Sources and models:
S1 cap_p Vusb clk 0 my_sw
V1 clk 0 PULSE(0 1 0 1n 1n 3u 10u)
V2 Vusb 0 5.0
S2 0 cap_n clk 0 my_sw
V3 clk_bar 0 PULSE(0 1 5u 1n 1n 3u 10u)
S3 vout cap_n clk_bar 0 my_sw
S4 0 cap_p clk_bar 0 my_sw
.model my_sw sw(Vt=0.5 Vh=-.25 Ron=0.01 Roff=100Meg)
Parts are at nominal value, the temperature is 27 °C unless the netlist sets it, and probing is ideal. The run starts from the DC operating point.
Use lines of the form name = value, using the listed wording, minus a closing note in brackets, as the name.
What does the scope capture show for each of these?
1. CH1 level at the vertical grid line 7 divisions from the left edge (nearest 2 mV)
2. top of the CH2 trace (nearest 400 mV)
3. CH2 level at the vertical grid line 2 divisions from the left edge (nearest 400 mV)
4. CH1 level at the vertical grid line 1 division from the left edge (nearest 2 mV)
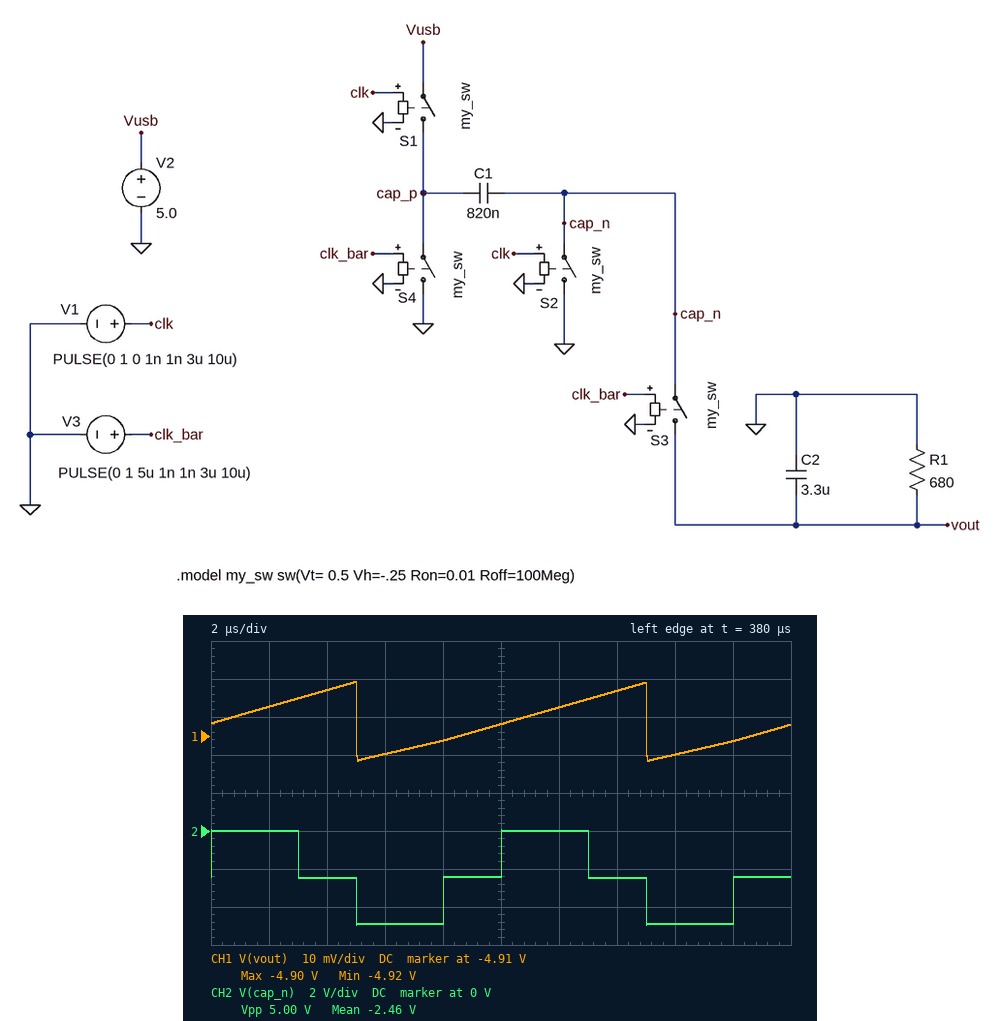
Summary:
CH1 level at the vertical grid line 7 divisions from the left edge = -4.898 V
top of the CH2 trace = 0 V
CH2 level at the vertical grid line 2 divisions from the left edge = -2.4 V
CH1 level at the vertical grid line 1 division from the left edge = -4.902 V
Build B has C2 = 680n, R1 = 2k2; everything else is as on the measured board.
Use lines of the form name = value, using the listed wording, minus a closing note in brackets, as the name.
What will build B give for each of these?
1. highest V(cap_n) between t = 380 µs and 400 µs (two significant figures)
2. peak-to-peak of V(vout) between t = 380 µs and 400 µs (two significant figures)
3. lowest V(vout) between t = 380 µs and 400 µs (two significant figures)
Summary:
highest V(cap_n) between t = 380 µs and 400 µs = 14 mV
peak-to-peak of V(vout) between t = 380 µs and 400 µs = 28 mV
lowest V(vout) between t = 380 µs and 400 µs = -5.0 V
